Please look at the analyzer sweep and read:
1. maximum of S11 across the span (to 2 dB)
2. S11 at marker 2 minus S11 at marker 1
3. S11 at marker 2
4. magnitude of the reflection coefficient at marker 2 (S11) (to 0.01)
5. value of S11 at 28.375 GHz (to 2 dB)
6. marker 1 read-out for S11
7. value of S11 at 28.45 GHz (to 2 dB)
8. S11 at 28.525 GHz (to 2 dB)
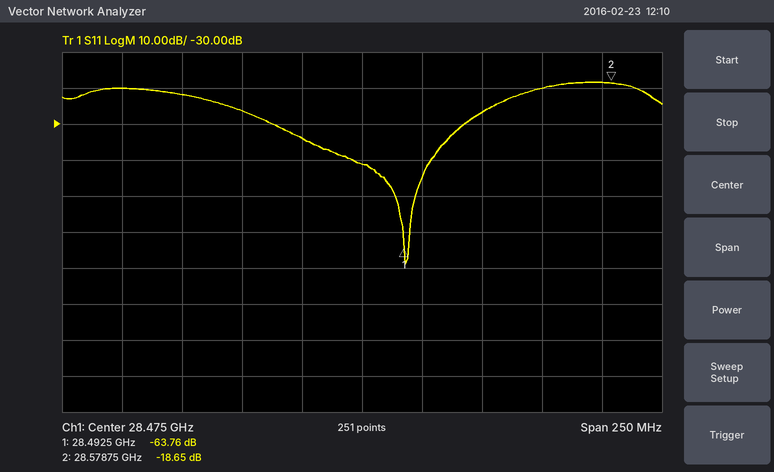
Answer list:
-18 dB
45.11 dB
-18.65 dB
0.12
-20 dB
-63.76 dB
-34 dB
-26 dB
